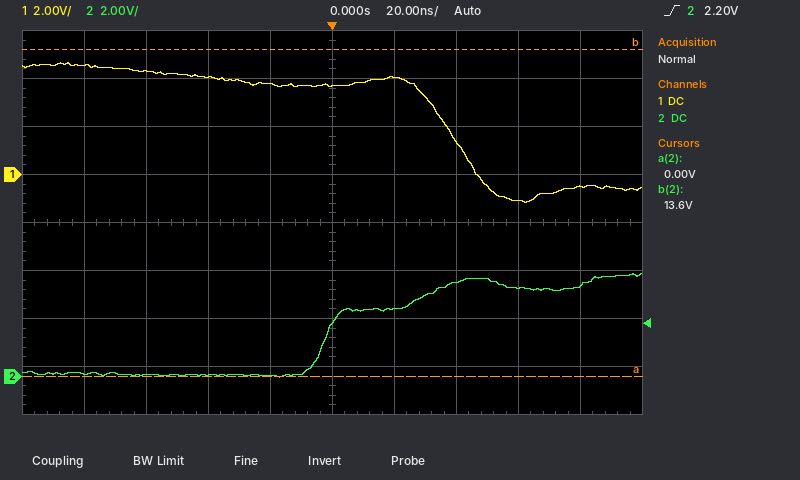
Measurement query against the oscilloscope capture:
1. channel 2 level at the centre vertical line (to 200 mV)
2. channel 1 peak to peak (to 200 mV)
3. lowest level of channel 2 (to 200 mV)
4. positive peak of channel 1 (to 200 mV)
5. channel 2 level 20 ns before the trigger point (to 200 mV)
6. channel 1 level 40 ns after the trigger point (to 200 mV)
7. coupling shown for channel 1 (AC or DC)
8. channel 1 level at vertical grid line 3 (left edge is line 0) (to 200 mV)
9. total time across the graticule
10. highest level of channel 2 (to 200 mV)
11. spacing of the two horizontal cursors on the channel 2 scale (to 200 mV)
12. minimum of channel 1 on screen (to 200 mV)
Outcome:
2.2 V
5.8 V
0.0 V
4.6 V
0.0 V
1.4 V
DC
4.0 V
200 ns
4.2 V
13.6 V
-1.2 V
